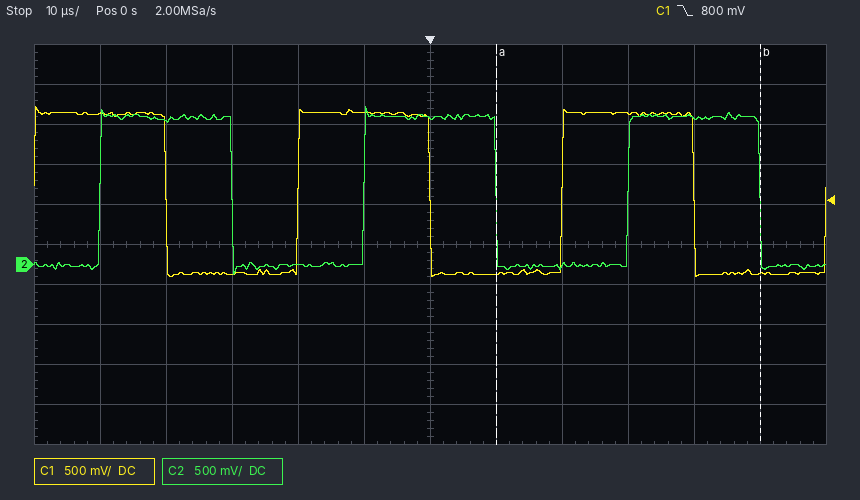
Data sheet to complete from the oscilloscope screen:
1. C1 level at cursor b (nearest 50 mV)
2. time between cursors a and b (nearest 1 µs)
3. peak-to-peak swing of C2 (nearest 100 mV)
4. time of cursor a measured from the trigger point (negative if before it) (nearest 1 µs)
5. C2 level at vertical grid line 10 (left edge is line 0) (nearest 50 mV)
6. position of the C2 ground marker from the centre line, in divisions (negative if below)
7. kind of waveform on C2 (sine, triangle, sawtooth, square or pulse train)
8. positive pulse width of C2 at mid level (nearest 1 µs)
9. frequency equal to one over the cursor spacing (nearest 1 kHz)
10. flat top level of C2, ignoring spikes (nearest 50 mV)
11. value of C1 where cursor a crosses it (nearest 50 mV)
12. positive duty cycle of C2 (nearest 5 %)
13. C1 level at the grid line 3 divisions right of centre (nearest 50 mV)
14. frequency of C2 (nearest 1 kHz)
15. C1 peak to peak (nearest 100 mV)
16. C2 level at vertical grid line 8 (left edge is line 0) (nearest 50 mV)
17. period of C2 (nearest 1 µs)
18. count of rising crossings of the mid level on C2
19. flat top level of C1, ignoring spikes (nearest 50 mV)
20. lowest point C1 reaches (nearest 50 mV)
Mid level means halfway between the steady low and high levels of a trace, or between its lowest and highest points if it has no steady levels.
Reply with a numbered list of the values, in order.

1. -100 mV
2. 40 µs
3. 2.10 V
4. +10 µs
5. 1.85 V
6. -0.5 div
7. square
8. 20 µs
9. 25 kHz
10. 1.85 V
11. -100 mV
12. 50 %
13. 1.90 V
14. 25 kHz
15. 2.10 V
16. 0 mV
17. 40 µs
18. 3
19. 1.90 V
20. -150 mV
